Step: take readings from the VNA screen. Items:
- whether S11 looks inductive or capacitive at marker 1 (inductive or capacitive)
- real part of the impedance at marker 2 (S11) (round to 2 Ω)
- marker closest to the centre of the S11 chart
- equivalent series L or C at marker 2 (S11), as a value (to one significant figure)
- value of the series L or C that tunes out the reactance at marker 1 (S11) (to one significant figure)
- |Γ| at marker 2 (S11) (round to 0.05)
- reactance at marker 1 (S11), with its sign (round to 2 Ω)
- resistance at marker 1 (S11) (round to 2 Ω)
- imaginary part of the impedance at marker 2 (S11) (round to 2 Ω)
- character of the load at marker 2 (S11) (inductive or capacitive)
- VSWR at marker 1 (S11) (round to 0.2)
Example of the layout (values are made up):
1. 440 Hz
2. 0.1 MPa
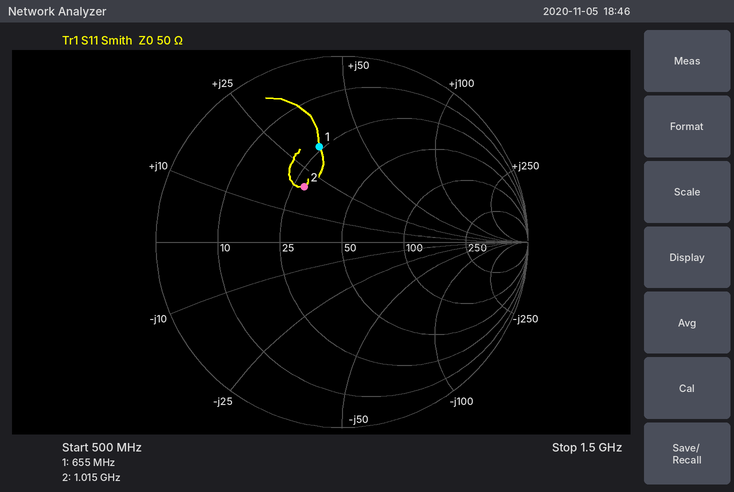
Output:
1. inductive
2. 28 Ω
3. marker 2
4. 3 nH
5. 7 pF
6. 0.35
7. +34 Ω
8. 24 Ω
9. +20 Ω
10. inductive
11. 3.2
